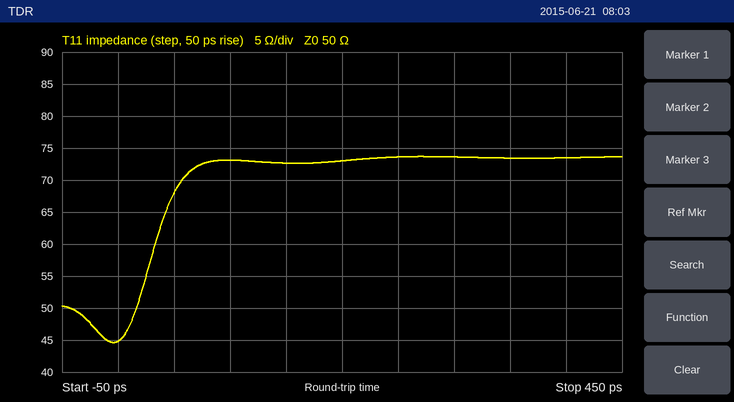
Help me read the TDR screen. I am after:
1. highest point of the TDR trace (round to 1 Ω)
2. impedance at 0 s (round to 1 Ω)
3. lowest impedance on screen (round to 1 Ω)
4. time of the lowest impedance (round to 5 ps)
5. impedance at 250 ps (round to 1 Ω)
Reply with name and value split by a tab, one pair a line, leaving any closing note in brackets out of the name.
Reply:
highest point of the TDR trace	74 Ω
impedance at 0 s	45 Ω
lowest impedance on screen	45 Ω
time of the lowest impedance	-5 ps
impedance at 250 ps	74 Ω
